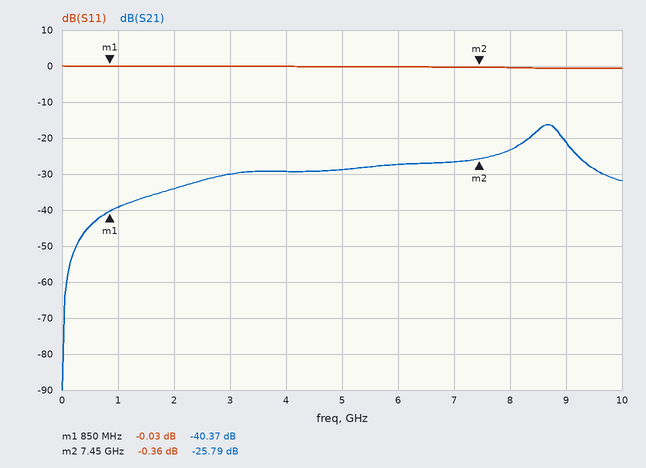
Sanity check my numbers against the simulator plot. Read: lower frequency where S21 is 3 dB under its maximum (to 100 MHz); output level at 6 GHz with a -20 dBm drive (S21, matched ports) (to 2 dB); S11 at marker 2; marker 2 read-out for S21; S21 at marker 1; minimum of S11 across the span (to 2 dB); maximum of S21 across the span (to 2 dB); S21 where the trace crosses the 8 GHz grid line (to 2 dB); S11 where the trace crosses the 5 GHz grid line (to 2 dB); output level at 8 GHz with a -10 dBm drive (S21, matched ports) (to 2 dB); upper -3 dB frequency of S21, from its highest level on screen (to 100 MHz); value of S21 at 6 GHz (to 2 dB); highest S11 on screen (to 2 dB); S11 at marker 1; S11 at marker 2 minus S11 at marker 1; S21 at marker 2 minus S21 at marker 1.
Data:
8.4 GHz
-48 dBm
-0.36 dB
-25.79 dB
-40.37 dB
0 dB
-16 dB
-24 dB
0 dB
-34 dBm
8.9 GHz
-28 dB
0 dB
-0.03 dB
-0.33 dB
14.58 dB
